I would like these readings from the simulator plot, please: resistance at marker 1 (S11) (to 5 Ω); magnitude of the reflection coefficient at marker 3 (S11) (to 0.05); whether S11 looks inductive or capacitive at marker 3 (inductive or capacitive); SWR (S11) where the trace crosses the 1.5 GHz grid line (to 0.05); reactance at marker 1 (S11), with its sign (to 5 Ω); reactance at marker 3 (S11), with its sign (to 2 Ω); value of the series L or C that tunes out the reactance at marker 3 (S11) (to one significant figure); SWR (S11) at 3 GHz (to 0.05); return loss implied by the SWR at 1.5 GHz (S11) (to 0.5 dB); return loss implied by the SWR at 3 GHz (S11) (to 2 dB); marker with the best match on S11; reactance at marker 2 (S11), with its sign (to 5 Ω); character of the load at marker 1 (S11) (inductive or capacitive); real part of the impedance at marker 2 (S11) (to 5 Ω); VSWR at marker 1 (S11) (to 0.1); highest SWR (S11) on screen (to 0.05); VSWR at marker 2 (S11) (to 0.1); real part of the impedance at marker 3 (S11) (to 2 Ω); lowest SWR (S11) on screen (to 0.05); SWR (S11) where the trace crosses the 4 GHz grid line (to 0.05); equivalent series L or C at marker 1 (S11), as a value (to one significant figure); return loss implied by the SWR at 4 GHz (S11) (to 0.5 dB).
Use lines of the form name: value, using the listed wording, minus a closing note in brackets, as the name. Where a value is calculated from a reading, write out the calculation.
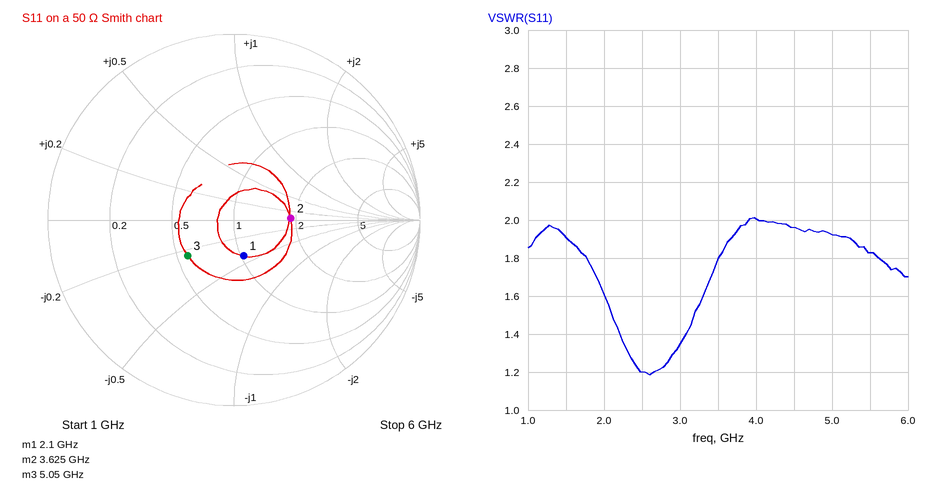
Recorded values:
resistance at marker 1 (S11): 50 Ω
magnitude of the reflection coefficient at marker 3 (S11): 0.30
whether S11 looks inductive or capacitive at marker 3: capacitive
SWR (S11) where the trace crosses the 1.5 GHz grid line: 1.90
reactance at marker 1 (S11), with its sign: -20 Ω
reactance at marker 3 (S11), with its sign: -12 Ω
value of the series L or C that tunes out the reactance at marker 3 (S11): L = 12 Ω/(2π × 5.05 GHz) ≈ 378 pH, so 400 pH to one significant figure
SWR (S11) at 3 GHz: 1.35
return loss implied by the SWR at 1.5 GHz (S11): −20 log10((1.9 − 1)/(1.9 + 1)) ≈ 10.2 dB, so 10.0 dB to the nearest 0.5 dB
return loss implied by the SWR at 3 GHz (S11): −20 log10((1.35 − 1)/(1.35 + 1)) ≈ 16 dB
marker with the best match on S11: marker 1
reactance at marker 2 (S11), with its sign: 0 Ω
character of the load at marker 1 (S11): capacitive
real part of the impedance at marker 2 (S11): 95 Ω
VSWR at marker 1 (S11): 1.5
highest SWR (S11) on screen: 2.00
VSWR at marker 2 (S11): 1.9
real part of the impedance at marker 3 (S11): 28 Ω
lowest SWR (S11) on screen: 1.20
SWR (S11) where the trace crosses the 4 GHz grid line: 2.00
equivalent series L or C at marker 1 (S11), as a value: C = 1/(2π × 2.1 GHz × 20 Ω) ≈ 4 pF
return loss implied by the SWR at 4 GHz (S11): −20 log10((2 − 1)/(2 + 1)) ≈ 9.5 dB
